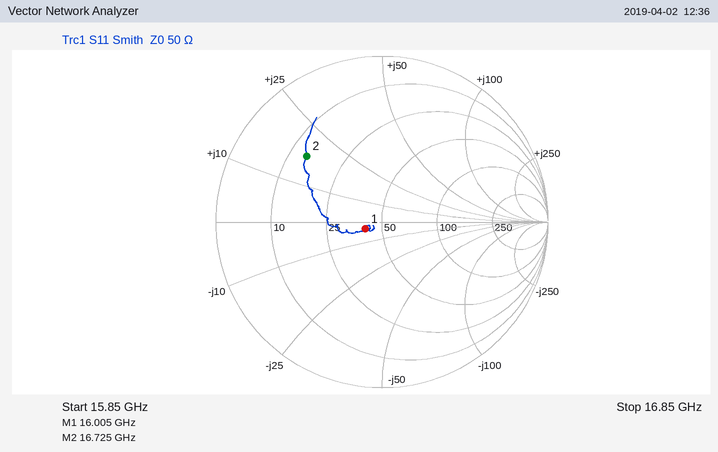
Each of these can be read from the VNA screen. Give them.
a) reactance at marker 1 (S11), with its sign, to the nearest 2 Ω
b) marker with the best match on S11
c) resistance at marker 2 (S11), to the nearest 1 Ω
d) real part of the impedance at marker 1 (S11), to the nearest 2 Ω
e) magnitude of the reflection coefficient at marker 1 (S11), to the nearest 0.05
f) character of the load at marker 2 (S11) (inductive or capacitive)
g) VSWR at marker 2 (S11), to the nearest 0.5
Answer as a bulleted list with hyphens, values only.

- -4 Ω
- marker 1
- 14 Ω
- 40 Ω
- 0.10
- inductive
- 4.0
